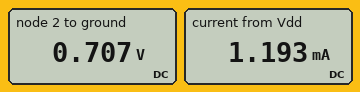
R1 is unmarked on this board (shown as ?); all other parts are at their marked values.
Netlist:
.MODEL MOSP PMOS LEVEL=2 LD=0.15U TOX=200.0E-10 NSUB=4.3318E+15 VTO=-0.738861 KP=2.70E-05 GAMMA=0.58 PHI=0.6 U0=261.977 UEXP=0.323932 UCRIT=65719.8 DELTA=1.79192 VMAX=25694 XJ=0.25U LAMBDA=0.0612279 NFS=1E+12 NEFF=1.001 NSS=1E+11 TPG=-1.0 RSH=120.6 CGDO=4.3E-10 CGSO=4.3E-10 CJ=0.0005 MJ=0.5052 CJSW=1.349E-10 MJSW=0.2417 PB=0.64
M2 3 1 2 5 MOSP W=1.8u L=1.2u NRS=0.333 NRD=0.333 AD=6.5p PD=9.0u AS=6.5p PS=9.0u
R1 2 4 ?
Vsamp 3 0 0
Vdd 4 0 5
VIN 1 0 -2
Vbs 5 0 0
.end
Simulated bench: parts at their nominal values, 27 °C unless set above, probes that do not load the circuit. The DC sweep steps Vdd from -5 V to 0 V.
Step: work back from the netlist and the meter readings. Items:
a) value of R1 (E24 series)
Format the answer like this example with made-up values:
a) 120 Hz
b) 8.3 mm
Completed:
a) 3.6 kΩ
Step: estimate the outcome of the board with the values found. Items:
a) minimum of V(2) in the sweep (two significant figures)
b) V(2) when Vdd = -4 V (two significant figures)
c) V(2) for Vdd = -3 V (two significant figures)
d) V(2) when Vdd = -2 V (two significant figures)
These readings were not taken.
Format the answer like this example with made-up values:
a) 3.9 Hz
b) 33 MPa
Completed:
a) -4.9 V
b) -3.9 V
c) -2.9 V
d) -1.9 V
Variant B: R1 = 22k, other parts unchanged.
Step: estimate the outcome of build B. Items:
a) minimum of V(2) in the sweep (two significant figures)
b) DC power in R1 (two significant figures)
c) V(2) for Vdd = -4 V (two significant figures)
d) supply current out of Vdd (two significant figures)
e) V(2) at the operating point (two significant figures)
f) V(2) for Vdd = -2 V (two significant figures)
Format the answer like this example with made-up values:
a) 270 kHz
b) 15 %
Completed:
a) -4.2 V
b) 870 µW
c) -3.3 V
d) 200 µA
e) 620 mV
f) -1.4 V
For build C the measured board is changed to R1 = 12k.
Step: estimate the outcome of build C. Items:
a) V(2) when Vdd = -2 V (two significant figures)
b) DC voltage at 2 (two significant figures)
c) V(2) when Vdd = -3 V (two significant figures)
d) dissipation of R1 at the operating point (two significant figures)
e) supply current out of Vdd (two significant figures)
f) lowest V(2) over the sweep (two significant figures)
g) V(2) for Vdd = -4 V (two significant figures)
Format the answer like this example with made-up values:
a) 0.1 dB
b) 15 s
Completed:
a) -1.7 V
b) 640 mV
c) -2.6 V
d) 1.6 mW
e) 360 µA
f) -4.6 V
g) -3.6 V
